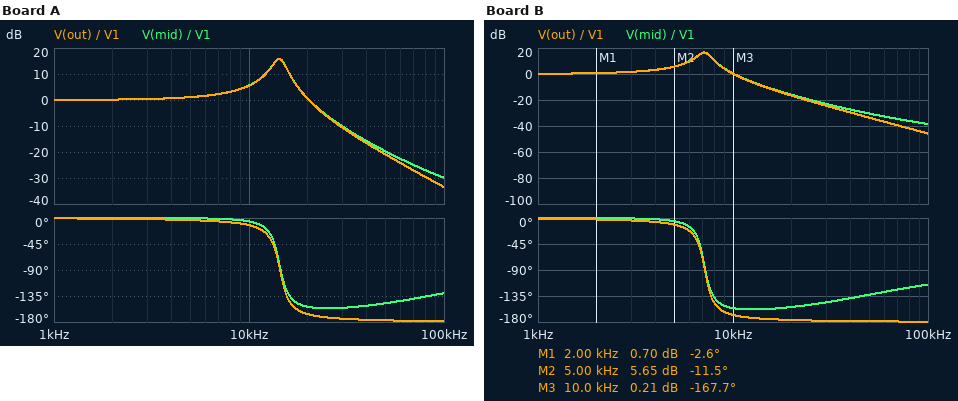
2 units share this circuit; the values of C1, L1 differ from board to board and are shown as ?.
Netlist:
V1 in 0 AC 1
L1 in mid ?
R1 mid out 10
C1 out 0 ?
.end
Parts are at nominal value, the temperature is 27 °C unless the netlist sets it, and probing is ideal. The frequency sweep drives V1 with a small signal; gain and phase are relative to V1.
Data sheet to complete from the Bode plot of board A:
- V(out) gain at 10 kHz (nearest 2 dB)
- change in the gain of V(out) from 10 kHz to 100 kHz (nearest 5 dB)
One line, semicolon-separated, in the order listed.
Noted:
6 dB; -40 dB
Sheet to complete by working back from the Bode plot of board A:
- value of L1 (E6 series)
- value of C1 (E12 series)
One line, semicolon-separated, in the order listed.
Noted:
680 µH; 180 nF
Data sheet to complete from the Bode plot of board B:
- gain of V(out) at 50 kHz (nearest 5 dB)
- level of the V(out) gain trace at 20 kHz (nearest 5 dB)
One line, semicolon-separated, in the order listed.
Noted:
-35 dB; -15 dB
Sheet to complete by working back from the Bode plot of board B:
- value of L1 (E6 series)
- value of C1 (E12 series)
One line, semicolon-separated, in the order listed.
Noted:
1.5 mH; 330 nF
